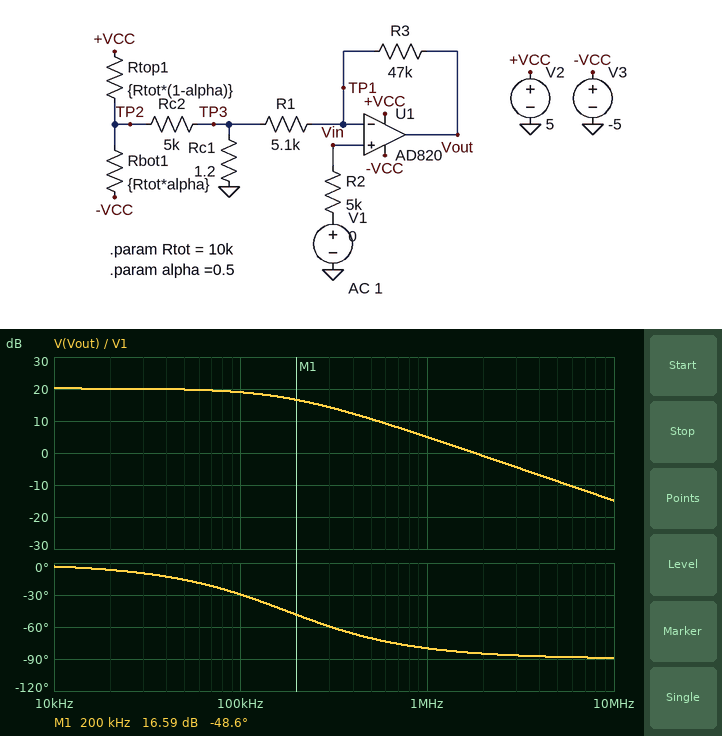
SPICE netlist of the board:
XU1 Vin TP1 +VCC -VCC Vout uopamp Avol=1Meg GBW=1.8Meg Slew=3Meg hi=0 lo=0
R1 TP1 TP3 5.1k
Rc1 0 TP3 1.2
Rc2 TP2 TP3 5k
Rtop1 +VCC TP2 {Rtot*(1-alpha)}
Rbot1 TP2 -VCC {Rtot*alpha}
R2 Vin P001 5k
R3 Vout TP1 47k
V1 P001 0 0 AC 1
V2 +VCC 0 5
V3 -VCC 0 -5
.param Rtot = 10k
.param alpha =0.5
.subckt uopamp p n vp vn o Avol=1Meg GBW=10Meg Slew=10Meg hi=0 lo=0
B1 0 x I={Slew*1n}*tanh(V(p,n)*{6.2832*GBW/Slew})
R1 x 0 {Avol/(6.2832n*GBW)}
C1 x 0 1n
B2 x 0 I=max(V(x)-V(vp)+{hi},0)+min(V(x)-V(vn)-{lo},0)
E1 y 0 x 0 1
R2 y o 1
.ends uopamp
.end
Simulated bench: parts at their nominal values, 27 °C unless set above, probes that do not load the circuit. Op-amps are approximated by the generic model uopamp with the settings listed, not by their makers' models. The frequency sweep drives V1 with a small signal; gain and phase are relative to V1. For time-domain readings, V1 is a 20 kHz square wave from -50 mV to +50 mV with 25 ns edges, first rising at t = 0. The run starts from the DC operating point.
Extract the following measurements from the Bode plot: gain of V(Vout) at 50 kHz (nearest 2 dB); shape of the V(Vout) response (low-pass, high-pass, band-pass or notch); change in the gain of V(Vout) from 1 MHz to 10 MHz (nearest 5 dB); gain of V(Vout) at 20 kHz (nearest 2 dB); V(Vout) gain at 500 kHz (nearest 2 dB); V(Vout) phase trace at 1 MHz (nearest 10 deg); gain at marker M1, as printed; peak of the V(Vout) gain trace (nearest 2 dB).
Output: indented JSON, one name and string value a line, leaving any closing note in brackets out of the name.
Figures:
{
  "gain of V(Vout) at 50 kHz": "20 dB",
  "shape of the V(Vout) response": "low-pass",
  "change in the gain of V(Vout) from 1 MHz to 10 MHz": "-20 dB",
  "gain of V(Vout) at 20 kHz": "20 dB",
  "V(Vout) gain at 500 kHz": "10 dB",
  "V(Vout) phase trace at 1 MHz": "-80 deg",
  "gain at marker M1, as printed": "16.59 dB",
  "peak of the V(Vout) gain trace": "20 dB"
}
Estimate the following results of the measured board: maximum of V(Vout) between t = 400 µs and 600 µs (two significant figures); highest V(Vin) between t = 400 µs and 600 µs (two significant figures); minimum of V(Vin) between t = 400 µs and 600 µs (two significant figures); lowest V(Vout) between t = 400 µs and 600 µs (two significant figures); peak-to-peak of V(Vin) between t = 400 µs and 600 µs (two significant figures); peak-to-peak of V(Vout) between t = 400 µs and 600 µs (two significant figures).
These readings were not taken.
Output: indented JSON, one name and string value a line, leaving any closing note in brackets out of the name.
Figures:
{
  "maximum of V(Vout) between t = 400 µs and 600 µs": "510 mV",
  "highest V(Vin) between t = 400 µs and 600 µs": "50 mV",
  "minimum of V(Vin) between t = 400 µs and 600 µs": "-50 mV",
  "lowest V(Vout) between t = 400 µs and 600 µs": "-510 mV",
  "peak-to-peak of V(Vin) between t = 400 µs and 600 µs": "100 mV",
  "peak-to-peak of V(Vout) between t = 400 µs and 600 µs": "1.0 V"
}
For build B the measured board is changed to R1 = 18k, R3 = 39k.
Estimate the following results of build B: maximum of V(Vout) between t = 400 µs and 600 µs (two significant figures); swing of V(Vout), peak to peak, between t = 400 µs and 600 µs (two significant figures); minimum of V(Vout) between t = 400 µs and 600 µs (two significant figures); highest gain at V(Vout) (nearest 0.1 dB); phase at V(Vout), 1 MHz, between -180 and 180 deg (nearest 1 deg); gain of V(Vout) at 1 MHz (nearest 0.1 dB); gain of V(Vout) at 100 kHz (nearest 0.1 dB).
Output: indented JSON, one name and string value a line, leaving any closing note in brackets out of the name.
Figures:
{
  "maximum of V(Vout) between t = 400 µs and 600 µs": "160 mV",
  "swing of V(Vout), peak to peak, between t = 400 µs and 600 µs": "320 mV",
  "minimum of V(Vout) between t = 400 µs and 600 µs": "-160 mV",
  "highest gain at V(Vout)": "10.0 dB",
  "phase at V(Vout), 1 MHz, between -180 and 180 deg": "-60 deg",
  "gain of V(Vout) at 1 MHz": "3.9 dB",
  "gain of V(Vout) at 100 kHz": "9.9 dB"
}
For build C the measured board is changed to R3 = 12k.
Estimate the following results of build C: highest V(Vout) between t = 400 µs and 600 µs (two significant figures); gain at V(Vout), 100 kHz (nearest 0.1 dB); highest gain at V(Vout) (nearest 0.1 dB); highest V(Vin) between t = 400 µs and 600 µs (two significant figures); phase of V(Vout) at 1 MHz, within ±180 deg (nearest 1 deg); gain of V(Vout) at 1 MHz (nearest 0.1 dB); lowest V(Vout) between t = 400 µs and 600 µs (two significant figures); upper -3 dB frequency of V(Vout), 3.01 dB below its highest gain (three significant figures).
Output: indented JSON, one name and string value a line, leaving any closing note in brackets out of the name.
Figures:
{
  "highest V(Vout) between t = 400 µs and 600 µs": "170 mV",
  "gain at V(Vout), 100 kHz": "10.4 dB",
  "highest gain at V(Vout)": "10.5 dB",
  "highest V(Vin) between t = 400 µs and 600 µs": "50 mV",
  "phase of V(Vout) at 1 MHz, within ±180 deg": "-62 deg",
  "gain of V(Vout) at 1 MHz": "4.0 dB",
  "lowest V(Vout) between t = 400 µs and 600 µs": "-170 mV",
  "upper -3 dB frequency of V(Vout), 3.01 dB below its highest gain": "537 kHz"
}
